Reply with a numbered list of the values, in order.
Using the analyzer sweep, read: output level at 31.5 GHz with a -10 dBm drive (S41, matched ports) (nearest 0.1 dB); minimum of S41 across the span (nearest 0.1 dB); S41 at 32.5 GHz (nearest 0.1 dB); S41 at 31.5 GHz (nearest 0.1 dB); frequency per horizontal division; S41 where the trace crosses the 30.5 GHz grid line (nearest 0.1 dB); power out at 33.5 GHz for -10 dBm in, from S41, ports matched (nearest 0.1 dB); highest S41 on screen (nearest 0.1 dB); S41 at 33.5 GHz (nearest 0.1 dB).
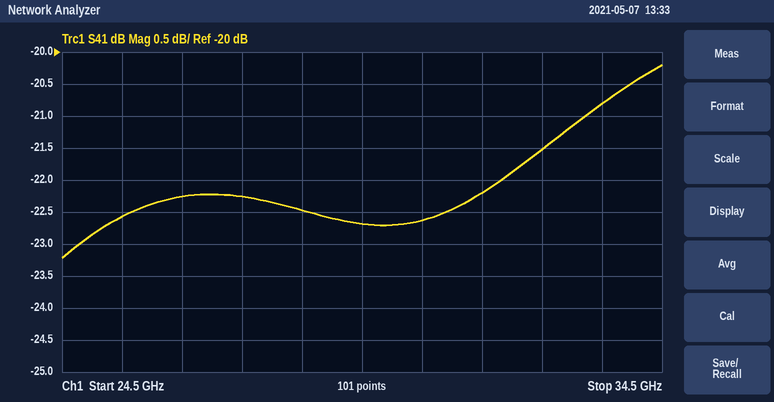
1. -32.2 dBm
2. -23.2 dB
3. -21.5 dB
4. -22.2 dB
5. 1 GHz
6. -22.6 dB
7. -30.8 dBm
8. -20.2 dB
9. -20.8 dB
